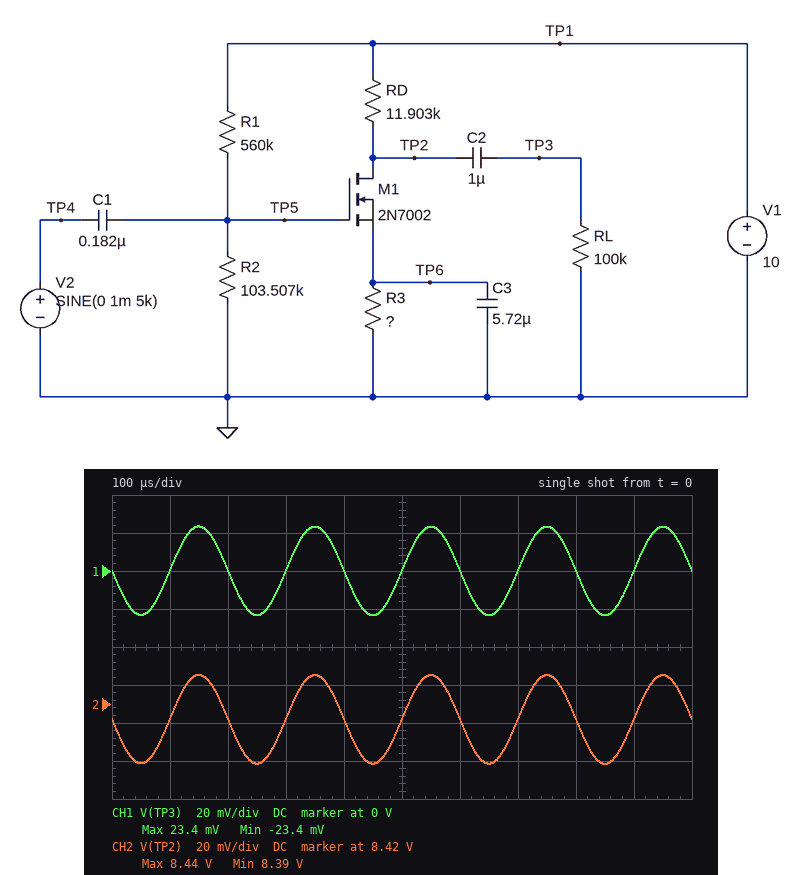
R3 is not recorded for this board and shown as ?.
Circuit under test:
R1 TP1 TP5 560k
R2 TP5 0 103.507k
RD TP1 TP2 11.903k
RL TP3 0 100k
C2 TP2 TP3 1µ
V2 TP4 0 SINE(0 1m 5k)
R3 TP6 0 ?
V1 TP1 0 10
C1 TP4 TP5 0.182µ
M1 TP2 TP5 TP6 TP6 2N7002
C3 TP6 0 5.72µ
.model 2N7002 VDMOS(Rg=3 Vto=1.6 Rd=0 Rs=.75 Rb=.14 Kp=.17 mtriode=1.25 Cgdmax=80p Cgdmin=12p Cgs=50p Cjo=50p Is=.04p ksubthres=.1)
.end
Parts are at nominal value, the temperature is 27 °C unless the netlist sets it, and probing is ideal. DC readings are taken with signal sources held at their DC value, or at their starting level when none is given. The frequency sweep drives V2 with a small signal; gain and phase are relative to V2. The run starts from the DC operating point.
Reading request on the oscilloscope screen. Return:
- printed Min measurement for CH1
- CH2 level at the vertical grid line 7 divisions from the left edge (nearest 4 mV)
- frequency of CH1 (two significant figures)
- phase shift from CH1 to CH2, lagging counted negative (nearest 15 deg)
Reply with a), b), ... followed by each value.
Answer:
a) -23.4 mV
b) 8.412 V
c) 5.0 kHz
d) 0 deg
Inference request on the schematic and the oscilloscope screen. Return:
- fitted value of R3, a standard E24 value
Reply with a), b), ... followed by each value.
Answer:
a) 240 Ω
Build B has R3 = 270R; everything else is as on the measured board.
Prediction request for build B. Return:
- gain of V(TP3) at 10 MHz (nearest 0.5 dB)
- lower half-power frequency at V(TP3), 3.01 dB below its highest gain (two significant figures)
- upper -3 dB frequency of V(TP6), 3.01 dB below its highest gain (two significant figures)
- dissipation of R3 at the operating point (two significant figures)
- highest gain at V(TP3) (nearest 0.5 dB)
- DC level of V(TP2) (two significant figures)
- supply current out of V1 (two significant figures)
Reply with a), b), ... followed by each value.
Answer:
a) 1.5 dB
b) 74 Hz
c) 180 Hz
d) 4.4 µW
e) 27.0 dB
f) 8.5 V
g) 140 µA
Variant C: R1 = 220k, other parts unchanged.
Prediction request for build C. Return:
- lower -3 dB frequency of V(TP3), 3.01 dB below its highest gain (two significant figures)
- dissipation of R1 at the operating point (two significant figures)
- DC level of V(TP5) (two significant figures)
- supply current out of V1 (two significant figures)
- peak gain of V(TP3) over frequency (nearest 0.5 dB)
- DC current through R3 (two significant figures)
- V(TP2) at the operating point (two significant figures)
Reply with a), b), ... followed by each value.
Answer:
a) 150 MHz
b) 210 µW
c) 3.2 V
d) 850 µA
e) -8.5 dB
f) 820 µA
g) 200 mV
